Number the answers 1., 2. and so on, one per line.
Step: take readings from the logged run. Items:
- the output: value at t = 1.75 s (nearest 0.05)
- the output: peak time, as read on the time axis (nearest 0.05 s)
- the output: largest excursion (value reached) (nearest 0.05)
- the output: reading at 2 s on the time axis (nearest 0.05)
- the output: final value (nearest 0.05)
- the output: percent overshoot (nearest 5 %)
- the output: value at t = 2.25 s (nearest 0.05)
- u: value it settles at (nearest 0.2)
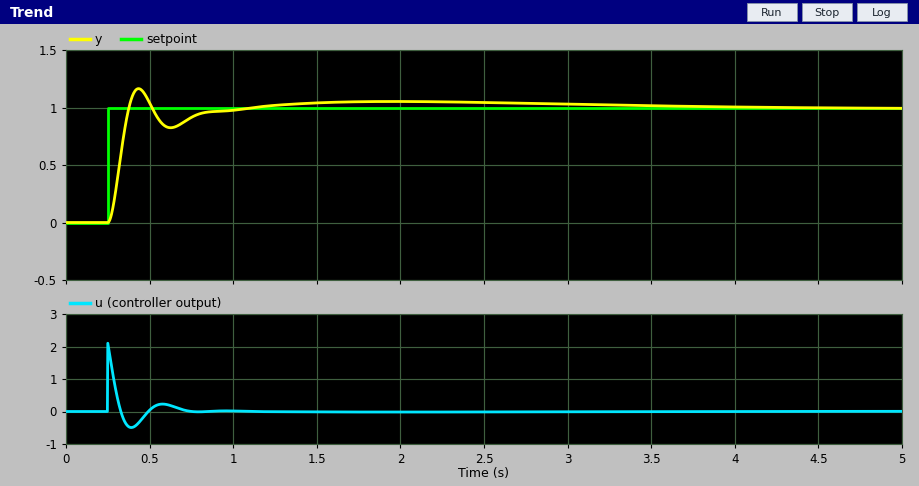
1. 1.05
2. 0.45 s
3. 1.15
4. 1.05
5. 1.00
6. 15 %
7. 1.05
8. 0.0
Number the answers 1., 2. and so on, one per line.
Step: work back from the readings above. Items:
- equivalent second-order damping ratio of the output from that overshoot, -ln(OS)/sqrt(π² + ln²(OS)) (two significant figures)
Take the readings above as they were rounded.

1. 0.52
